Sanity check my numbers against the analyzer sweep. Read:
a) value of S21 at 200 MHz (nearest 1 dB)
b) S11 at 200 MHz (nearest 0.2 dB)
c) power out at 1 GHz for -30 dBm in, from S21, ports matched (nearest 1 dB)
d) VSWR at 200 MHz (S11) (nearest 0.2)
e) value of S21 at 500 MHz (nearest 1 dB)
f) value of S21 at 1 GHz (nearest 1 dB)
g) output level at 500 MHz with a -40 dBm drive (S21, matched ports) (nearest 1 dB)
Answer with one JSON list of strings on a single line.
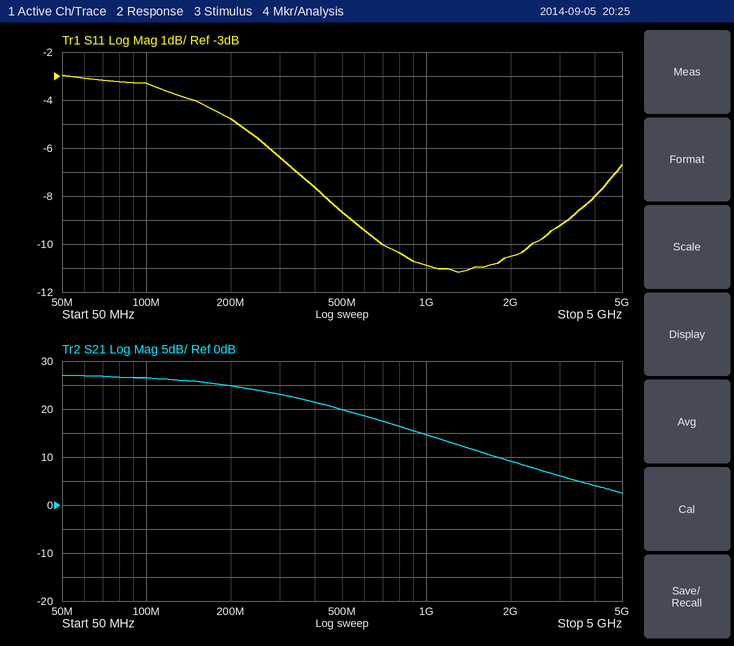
["25 dB", "-4.8 dB", "-15 dBm", "3.8", "20 dB", "15 dB", "-20 dBm"]
